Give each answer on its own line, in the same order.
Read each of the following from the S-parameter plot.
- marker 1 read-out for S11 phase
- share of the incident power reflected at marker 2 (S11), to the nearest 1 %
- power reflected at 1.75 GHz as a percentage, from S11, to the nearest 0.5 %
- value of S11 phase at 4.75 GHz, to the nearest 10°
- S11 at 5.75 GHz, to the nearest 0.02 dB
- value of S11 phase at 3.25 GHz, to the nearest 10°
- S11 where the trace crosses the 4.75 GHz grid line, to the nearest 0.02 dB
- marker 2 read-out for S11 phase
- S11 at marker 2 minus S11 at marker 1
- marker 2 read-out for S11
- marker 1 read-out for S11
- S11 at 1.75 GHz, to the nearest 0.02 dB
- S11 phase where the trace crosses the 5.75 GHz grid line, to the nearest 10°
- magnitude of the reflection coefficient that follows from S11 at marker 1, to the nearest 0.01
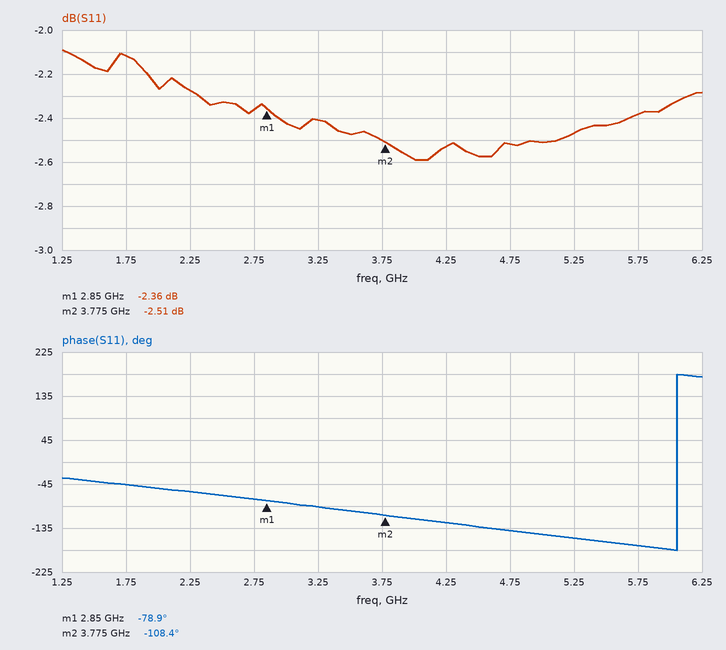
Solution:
-78.9°
56 %
61.5 %
-140°
-2.38 dB
-90°
-2.52 dB
-108.4°
-0.15 dB
-2.51 dB
-2.36 dB
-2.12 dB
-170°
0.76
